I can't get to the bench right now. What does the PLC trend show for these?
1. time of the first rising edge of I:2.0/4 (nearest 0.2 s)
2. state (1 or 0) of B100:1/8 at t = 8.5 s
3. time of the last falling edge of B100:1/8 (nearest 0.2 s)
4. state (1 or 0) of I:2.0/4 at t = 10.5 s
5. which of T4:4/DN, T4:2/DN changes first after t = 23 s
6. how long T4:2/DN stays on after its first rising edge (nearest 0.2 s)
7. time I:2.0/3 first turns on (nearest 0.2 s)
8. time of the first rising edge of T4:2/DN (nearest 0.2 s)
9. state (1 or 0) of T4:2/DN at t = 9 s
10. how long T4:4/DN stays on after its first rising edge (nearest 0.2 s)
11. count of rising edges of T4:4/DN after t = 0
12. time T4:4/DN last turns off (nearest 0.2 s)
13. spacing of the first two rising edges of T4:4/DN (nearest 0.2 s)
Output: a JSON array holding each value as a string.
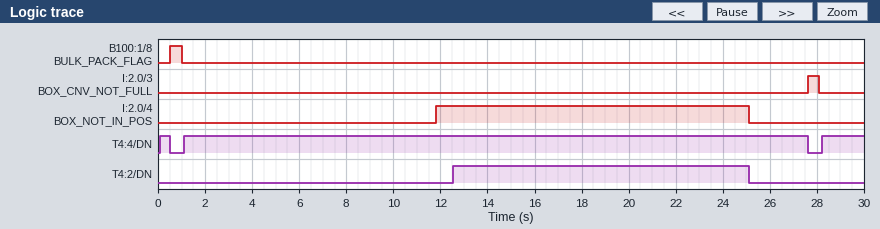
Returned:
["11.8 s", "0", "1.0 s", "0", "T4:2/DN", "12.6 s", "27.6 s", "12.6 s", "0", "0.4 s", "3", "27.6 s", "1.0 s"]
